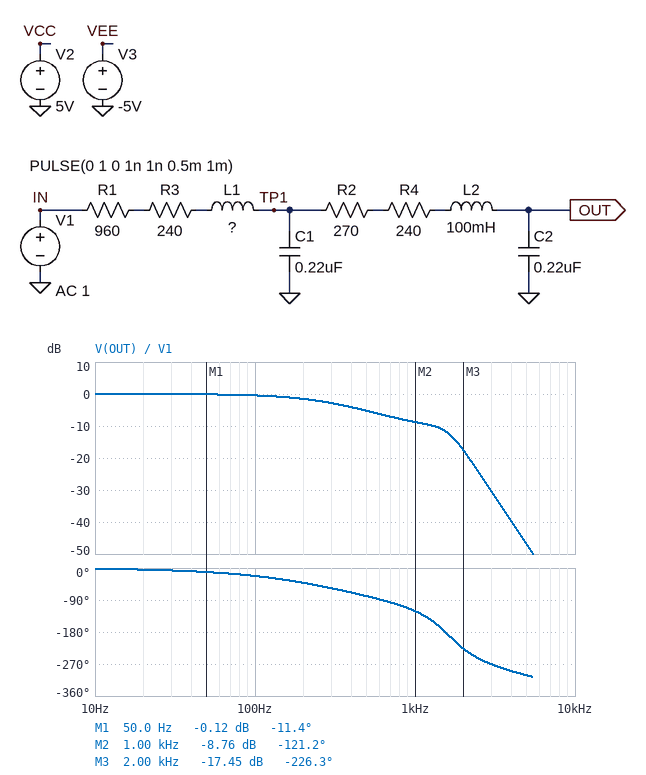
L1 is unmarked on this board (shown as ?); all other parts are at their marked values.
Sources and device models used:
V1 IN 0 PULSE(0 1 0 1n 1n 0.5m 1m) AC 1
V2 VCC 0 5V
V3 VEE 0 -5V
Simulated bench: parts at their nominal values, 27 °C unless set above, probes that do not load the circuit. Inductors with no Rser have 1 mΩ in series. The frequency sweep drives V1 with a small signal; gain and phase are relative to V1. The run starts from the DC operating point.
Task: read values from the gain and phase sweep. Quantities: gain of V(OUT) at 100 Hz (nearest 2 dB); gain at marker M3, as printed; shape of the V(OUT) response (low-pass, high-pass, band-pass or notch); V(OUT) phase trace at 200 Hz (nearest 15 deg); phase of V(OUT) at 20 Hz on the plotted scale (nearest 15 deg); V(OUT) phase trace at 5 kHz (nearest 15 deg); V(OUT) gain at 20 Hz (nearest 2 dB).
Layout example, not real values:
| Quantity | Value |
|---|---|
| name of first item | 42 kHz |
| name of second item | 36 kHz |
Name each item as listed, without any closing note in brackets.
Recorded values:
| Quantity | Value |
|---|---|
| gain of V(OUT) at 100 Hz | 0 dB |
| gain at marker M3, as printed | -17.45 dB |
| shape of the V(OUT) response | low-pass |
| V(OUT) phase trace at 200 Hz | -45 deg |
| phase of V(OUT) at 20 Hz on the plotted scale | 0 deg |
| V(OUT) phase trace at 5 kHz | -300 deg |
| V(OUT) gain at 20 Hz | 0 dB |
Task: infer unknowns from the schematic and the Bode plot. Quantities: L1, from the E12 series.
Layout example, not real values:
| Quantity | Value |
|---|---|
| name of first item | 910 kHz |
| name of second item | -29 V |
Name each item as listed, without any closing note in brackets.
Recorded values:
| Quantity | Value |
|---|---|
| L1, from the E12 series | 39 mH |
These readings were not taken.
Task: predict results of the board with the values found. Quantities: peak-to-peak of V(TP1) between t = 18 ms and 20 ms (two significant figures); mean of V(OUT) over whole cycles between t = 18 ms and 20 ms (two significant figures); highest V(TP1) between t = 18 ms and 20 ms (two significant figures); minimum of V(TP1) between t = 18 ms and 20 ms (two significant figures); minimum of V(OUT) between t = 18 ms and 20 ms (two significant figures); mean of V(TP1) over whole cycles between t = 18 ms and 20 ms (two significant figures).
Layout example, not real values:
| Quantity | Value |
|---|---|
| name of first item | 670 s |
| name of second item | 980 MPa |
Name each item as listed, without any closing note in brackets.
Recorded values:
| Quantity | Value |
|---|---|
| peak-to-peak of V(TP1) between t = 18 ms and 20 ms | 340 mV |
| mean of V(OUT) over whole cycles between t = 18 ms and 20 ms | 500 mV |
| highest V(TP1) between t = 18 ms and 20 ms | 670 mV |
| minimum of V(TP1) between t = 18 ms and 20 ms | 330 mV |
| minimum of V(OUT) between t = 18 ms and 20 ms | 270 mV |
| mean of V(TP1) over whole cycles between t = 18 ms and 20 ms | 500 mV |
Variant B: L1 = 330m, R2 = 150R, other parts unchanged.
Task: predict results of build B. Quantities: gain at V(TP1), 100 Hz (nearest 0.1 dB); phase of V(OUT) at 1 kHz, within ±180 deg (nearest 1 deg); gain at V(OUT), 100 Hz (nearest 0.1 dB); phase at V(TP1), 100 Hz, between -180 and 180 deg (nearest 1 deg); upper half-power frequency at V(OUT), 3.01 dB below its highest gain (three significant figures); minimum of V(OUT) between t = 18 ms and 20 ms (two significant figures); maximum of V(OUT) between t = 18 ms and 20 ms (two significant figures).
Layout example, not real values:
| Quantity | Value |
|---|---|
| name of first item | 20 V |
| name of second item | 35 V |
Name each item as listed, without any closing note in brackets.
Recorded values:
| Quantity | Value |
|---|---|
| gain at V(TP1), 100 Hz | -0.1 dB |
| phase of V(OUT) at 1 kHz, within ±180 deg | -168 deg |
| gain at V(OUT), 100 Hz | 0 dB |
| phase at V(TP1), 100 Hz, between -180 and 180 deg | -19 deg |
| upper half-power frequency at V(OUT), 3.01 dB below its highest gain | 418 Hz |
| minimum of V(OUT) between t = 18 ms and 20 ms | 340 mV |
| maximum of V(OUT) between t = 18 ms and 20 ms | 660 mV |
